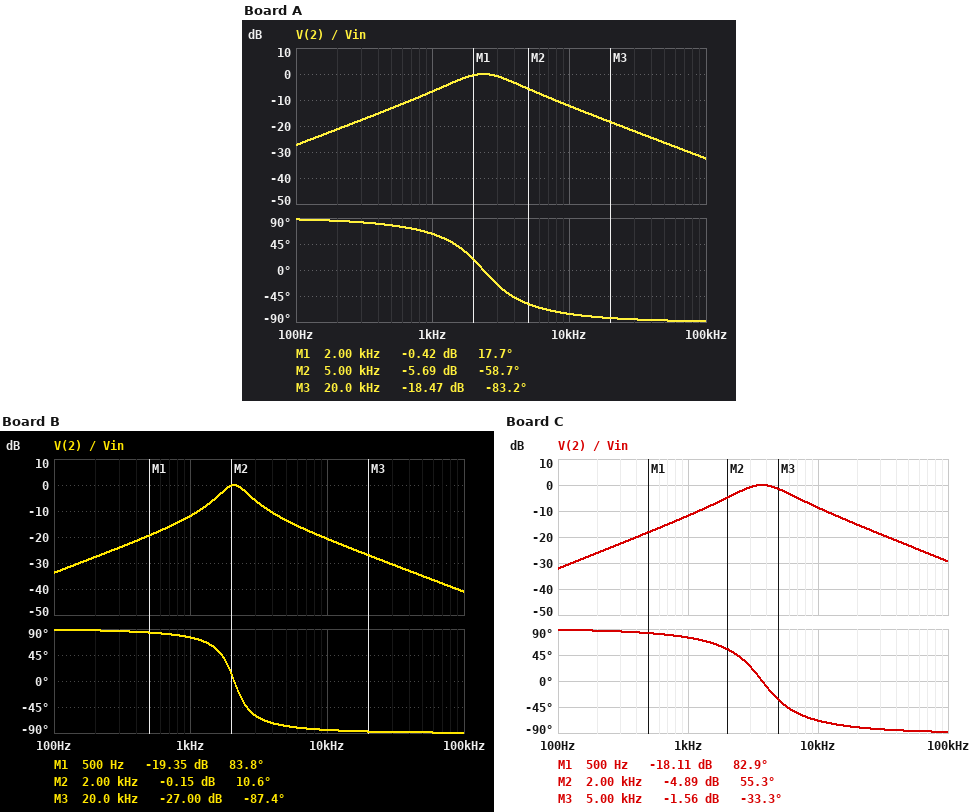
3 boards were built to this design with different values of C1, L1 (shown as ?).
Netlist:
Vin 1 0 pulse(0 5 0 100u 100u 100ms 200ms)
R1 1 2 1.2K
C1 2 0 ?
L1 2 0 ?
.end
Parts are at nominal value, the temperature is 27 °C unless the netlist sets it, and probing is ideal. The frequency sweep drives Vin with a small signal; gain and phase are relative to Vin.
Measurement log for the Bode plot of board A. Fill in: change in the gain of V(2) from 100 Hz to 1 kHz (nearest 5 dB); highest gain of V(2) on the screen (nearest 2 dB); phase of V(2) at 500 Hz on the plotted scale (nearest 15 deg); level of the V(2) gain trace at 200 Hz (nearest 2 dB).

20 dB
0 dB
75 deg
-22 dB
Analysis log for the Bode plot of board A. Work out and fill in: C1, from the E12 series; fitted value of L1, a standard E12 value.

56 nF
82 mH
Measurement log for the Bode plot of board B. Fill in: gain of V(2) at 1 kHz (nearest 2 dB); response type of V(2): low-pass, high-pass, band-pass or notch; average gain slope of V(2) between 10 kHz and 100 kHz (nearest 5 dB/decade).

-12 dB
band-pass
-20 dB/decade
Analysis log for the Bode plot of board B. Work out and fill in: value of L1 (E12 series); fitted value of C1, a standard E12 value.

39 mH
150 nF
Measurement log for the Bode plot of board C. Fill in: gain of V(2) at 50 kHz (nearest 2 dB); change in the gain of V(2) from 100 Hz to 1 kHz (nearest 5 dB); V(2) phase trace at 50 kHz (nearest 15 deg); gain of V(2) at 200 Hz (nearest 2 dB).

-24 dB
20 dB
-90 deg
-26 dB
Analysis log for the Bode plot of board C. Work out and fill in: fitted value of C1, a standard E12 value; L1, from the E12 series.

39 nF
47 mH
